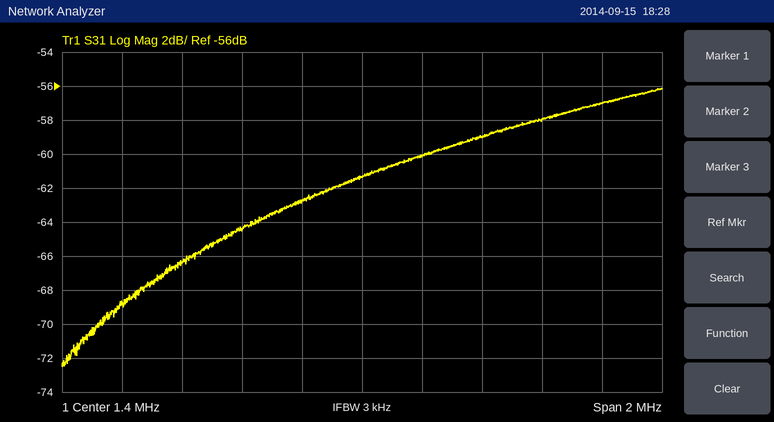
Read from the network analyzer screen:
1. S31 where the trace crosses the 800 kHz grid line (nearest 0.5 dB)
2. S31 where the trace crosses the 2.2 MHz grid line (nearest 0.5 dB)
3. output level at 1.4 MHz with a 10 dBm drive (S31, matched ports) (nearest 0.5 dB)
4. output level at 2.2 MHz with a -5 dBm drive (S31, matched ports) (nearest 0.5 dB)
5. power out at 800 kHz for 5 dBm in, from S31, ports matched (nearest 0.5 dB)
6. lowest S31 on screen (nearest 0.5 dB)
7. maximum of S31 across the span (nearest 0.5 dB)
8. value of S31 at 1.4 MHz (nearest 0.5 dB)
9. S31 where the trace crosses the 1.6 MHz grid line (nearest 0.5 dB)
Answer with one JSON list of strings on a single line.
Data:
["-66.5 dB", "-57.0 dB", "-51.5 dBm", "-62.0 dBm", "-61.5 dBm", "-72.5 dB", "-56.0 dB", "-61.5 dB", "-60.0 dB"]
